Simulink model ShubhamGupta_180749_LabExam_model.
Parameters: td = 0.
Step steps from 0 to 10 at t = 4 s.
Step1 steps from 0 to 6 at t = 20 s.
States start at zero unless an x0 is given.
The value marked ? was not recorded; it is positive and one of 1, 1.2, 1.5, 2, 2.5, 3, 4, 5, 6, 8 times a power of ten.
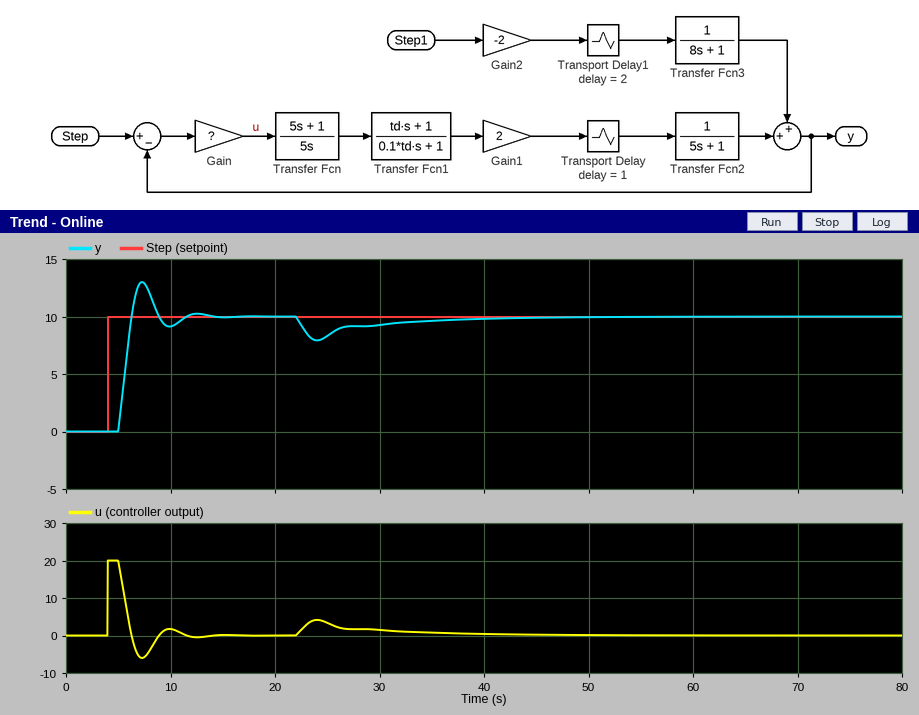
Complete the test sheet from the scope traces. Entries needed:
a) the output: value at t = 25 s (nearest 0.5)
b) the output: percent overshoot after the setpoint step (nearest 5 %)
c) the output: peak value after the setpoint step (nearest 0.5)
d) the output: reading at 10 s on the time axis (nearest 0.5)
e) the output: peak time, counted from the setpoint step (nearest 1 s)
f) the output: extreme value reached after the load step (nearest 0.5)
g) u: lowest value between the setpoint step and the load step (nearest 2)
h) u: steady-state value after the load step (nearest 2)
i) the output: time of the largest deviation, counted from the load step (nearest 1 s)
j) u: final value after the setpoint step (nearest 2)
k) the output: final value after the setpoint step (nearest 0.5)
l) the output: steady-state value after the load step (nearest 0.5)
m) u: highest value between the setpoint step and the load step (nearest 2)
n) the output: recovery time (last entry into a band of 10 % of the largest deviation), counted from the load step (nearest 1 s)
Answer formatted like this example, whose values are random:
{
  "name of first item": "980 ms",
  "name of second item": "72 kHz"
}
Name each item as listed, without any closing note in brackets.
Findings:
{
  "the output: value at t = 25 s": "8.5",
  "the output: percent overshoot after the setpoint step": "30 %",
  "the output: peak value after the setpoint step": "13.0",
  "the output: reading at 10 s on the time axis": "9.0",
  "the output: peak time, counted from the setpoint step": "3 s",
  "the output: extreme value reached after the load step": "8.0",
  "u: lowest value between the setpoint step and the load step": "-6",
  "u: steady-state value after the load step": "0",
  "the output: time of the largest deviation, counted from the load step": "4 s",
  "u: final value after the setpoint step": "0",
  "the output: final value after the setpoint step": "10.0",
  "the output: steady-state value after the load step": "10.0",
  "u: highest value between the setpoint step and the load step": "20",
  "the output: recovery time (last entry into a band of 10 % of the largest deviation), counted from the load step": "20 s"
}
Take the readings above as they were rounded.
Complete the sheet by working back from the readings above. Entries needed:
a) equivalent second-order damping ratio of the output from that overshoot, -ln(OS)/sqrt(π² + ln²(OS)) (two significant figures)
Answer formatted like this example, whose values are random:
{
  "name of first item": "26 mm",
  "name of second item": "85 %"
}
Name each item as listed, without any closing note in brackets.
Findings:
{
  "equivalent second-order damping ratio of the output from that overshoot, -ln(OS)/sqrt(π² + ln²(OS))": "0.36"
}
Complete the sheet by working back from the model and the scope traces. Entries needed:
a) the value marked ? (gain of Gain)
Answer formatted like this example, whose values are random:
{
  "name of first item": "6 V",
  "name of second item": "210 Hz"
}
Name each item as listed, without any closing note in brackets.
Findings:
{
  "the value marked ?": "2"
}
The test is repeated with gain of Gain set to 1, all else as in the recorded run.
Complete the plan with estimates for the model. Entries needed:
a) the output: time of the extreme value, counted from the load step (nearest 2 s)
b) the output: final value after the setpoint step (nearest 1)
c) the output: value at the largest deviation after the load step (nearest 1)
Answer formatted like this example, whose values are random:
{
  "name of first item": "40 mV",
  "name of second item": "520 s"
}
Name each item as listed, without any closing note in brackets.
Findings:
{
  "the output: time of the extreme value, counted from the load step": "6 s",
  "the output: final value after the setpoint step": "10",
  "the output: value at the largest deviation after the load step": "7"
}
